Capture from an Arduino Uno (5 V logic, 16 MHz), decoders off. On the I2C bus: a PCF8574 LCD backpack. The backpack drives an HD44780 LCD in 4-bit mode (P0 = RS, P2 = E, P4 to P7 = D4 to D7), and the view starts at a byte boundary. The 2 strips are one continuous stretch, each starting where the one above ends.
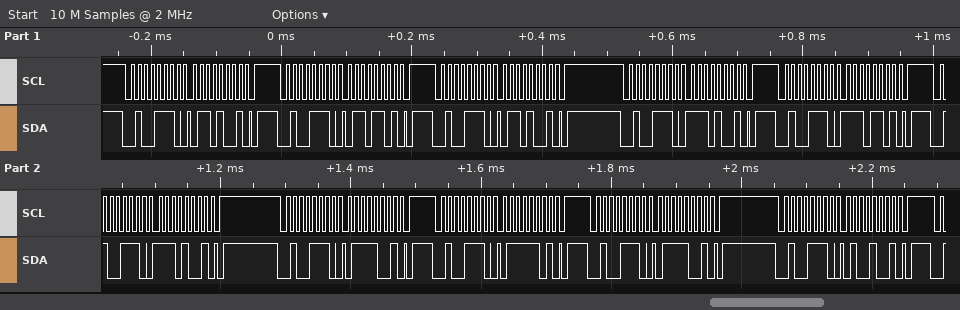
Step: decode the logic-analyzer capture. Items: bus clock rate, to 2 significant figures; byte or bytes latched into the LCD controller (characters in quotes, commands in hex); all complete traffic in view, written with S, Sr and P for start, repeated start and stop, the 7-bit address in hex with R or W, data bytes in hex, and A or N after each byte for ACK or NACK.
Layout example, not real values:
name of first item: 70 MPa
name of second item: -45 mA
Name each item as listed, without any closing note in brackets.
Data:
bus clock rate, to 2 significant figures: 100 kHz
byte or bytes latched into the LCD controller: 'n'
all complete traffic in view, written with S, Sr and P for start, repeated start and stop, the 7-bit address in hex with R or W, data bytes in hex, and A or N after each byte for ACK or NACK: S 27W A 69 A P S 27W A 6D A P S 27W A 69 A P S 27W A E9 A P S 27W A ED A P S 27W A E9 A P S 27W A 79 A P S 27W A 7D A P S 27W A 79 A P S 27W A 49 A P
